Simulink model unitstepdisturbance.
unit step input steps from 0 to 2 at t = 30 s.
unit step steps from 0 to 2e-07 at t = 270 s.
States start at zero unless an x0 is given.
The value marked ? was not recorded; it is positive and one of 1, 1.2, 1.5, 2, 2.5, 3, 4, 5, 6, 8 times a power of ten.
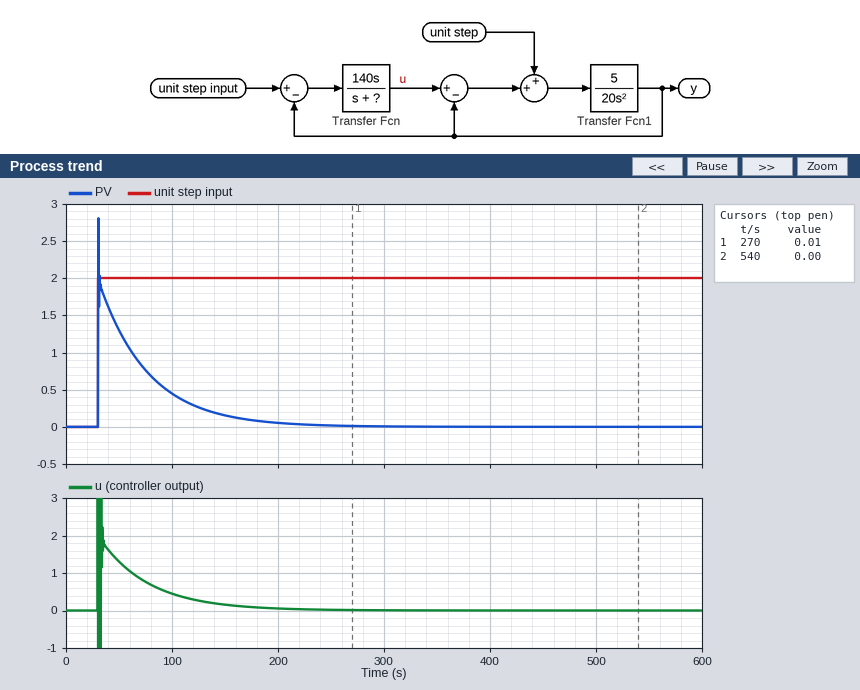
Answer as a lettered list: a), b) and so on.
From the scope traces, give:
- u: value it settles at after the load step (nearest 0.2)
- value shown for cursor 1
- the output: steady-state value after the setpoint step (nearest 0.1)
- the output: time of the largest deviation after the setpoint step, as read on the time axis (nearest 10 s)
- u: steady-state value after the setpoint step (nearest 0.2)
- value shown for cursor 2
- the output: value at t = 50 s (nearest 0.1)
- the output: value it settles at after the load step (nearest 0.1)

a) 0.0
b) 0.01
c) 0.0
d) 30 s
e) 0.0
f) 0.00
g) 1.3
h) 0.0
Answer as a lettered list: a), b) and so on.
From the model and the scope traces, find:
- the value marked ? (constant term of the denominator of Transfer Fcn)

a) 3
